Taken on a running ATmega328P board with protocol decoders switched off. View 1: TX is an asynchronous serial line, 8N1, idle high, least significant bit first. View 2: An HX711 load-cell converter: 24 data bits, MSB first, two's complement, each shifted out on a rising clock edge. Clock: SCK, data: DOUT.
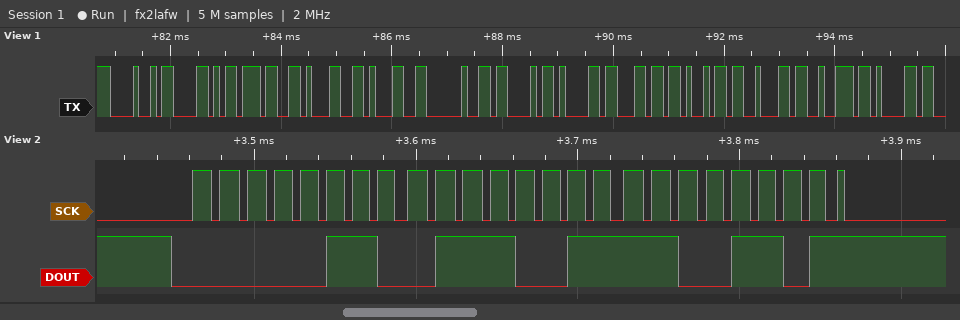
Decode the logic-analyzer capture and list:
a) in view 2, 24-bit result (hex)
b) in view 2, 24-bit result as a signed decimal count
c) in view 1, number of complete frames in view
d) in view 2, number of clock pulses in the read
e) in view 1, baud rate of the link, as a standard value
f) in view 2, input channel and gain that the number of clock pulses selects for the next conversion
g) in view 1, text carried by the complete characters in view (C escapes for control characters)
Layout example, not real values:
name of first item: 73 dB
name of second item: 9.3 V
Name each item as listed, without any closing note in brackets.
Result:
in view 2, 24-bit result: 0x0673CD
in view 2, 24-bit result as a signed decimal count: 422861
in view 1, number of complete frames in view: 13
in view 2, number of clock pulses in the read: 25
in view 1, baud rate of the link, as a standard value: 9600 baud
in view 2, input channel and gain that the number of clock pulses selects for the next conversion: channel A, gain 128
in view 1, text carried by the complete characters in view: "HX711 Calibra"
